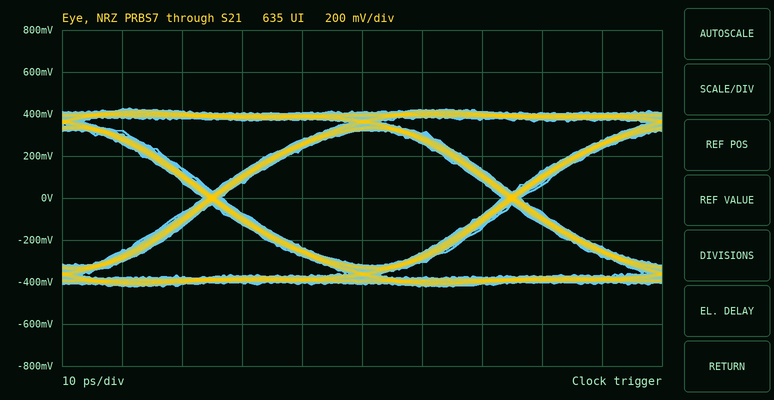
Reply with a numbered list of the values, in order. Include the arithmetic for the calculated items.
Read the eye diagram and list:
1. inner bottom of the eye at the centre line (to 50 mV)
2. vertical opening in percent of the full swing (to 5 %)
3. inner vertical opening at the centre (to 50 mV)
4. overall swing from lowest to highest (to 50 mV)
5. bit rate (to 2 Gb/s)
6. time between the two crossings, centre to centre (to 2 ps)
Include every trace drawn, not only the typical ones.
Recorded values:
1. -300 mV
2. 650 mV / 850 mV ≈ 76.5 %, so 75 % to the nearest 5 %
3. 650 mV
4. 850 mV
5. 20 Gb/s
6. 50 ps
